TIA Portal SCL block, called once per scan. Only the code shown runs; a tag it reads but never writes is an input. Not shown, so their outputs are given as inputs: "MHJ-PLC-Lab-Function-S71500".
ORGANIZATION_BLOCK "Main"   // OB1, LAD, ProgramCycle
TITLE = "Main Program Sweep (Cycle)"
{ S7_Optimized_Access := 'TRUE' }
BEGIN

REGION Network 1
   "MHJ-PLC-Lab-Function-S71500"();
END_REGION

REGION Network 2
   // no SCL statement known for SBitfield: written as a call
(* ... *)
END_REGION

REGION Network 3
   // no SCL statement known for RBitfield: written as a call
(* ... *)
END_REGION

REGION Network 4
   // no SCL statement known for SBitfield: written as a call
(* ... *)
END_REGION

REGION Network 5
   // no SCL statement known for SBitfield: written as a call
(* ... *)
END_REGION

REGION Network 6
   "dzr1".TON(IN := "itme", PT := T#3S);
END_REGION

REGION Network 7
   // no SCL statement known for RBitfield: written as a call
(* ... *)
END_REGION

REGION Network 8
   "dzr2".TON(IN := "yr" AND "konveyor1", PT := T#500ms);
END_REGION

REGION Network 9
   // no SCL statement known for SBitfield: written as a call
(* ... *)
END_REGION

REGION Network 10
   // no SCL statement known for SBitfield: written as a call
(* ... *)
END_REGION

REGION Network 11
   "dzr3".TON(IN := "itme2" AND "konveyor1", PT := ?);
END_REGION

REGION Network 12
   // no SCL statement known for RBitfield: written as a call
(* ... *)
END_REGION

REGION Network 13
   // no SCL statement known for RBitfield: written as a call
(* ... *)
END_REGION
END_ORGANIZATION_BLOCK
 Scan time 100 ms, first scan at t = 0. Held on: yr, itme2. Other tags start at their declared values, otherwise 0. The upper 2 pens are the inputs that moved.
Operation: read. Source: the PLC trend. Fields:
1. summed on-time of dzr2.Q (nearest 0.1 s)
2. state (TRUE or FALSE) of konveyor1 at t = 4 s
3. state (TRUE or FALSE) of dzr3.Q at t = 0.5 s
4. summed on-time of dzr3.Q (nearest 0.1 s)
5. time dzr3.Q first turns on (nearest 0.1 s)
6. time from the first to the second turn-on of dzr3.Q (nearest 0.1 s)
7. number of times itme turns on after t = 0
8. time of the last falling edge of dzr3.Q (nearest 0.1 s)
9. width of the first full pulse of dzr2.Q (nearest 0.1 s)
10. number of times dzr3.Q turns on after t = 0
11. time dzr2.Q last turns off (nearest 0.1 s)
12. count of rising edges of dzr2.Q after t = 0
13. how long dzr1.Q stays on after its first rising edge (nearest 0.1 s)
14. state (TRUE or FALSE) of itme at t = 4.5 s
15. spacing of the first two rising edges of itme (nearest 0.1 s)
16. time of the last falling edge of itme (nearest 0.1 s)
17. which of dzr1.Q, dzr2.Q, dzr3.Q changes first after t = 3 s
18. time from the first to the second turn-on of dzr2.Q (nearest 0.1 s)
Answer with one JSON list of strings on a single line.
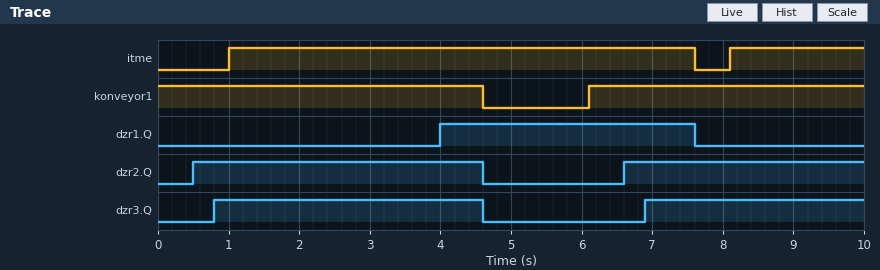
["7.5 s", "TRUE", "FALSE", "6.9 s", "0.8 s", "6.1 s", "2", "4.6 s", "4.1 s", "2", "4.6 s", "2", "3.6 s", "TRUE", "7.1 s", "7.6 s", "dzr1.Q", "6.1 s"]
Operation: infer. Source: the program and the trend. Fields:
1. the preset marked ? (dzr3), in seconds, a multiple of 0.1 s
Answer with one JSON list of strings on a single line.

["0.8 s"]
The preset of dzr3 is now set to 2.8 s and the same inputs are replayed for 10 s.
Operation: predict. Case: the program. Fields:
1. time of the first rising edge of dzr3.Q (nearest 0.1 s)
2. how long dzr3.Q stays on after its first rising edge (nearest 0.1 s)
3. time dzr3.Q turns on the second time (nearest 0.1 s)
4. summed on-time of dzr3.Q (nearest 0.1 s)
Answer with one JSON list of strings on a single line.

["2.8 s", "1.8 s", "8.9 s", "2.9 s"]
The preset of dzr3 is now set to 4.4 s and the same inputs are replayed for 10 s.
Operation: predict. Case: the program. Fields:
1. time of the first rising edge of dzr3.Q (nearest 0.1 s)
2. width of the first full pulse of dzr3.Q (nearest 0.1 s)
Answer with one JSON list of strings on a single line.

["4.4 s", "0.2 s"]
